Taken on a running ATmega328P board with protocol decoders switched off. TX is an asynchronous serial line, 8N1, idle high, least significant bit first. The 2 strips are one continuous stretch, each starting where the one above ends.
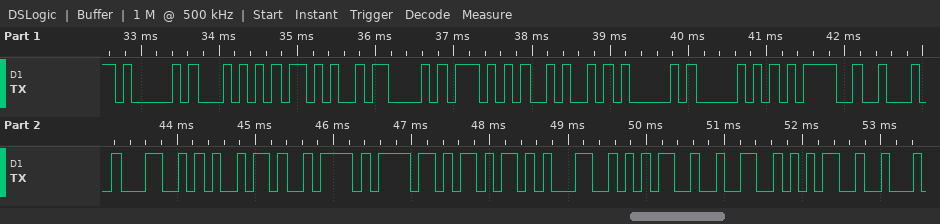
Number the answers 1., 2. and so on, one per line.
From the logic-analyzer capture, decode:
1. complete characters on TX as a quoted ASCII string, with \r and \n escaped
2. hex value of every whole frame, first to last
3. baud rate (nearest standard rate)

1. "AT+CWJAP=\"Lizok1525"
2. 41 54 2B 43 57 4A 41 50 3D 22 4C 69 7A 6F 6B 31 35 32 35
3. 9600 baud
